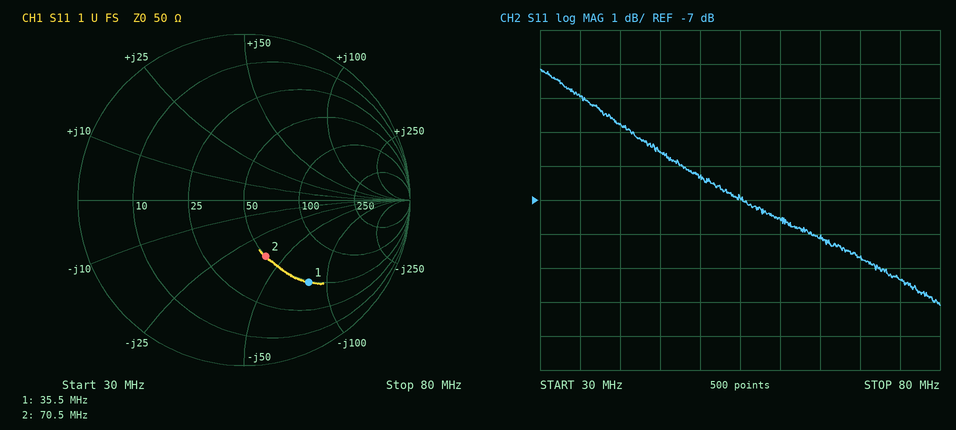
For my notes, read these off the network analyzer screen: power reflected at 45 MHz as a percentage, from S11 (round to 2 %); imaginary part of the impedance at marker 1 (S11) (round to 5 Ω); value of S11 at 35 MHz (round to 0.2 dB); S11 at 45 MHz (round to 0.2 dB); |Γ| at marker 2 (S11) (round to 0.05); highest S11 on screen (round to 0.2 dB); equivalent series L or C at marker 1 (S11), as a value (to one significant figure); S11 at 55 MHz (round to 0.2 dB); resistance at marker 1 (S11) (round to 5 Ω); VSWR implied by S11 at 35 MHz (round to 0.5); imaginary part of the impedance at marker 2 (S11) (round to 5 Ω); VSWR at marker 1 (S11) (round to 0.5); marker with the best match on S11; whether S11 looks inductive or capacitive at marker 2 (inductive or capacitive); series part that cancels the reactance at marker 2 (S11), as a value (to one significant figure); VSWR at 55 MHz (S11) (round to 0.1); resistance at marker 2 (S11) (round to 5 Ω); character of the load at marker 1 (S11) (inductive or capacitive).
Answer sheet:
28 %
-80 Ω
-4.0 dB
-5.6 dB
0.35
-3.2 dB
60 pF
-7.0 dB
50 Ω
4.5
-40 Ω
4.5
marker 2
capacitive
90 nH
2.6
50 Ω
capacitive
